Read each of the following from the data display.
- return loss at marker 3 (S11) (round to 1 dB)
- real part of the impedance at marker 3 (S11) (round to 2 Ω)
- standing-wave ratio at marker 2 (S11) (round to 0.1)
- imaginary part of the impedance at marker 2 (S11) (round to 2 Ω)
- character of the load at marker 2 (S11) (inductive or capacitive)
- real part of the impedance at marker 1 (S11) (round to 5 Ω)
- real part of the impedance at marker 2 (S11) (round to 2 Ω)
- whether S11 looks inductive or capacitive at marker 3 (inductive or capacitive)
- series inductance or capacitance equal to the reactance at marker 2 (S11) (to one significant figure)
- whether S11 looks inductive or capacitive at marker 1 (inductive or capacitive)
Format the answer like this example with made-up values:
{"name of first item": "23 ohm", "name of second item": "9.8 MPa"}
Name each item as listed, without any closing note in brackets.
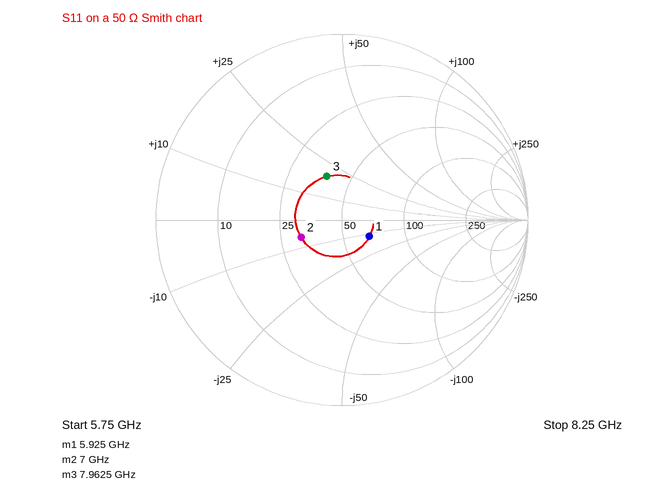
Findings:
{"return loss at marker 3 (S11)": "12 dB", "real part of the impedance at marker 3 (S11)": "38 Ω", "standing-wave ratio at marker 2 (S11)": "1.6", "imaginary part of the impedance at marker 2 (S11)": "-6 Ω", "character of the load at marker 2 (S11)": "capacitive", "real part of the impedance at marker 1 (S11)": "65 Ω", "real part of the impedance at marker 2 (S11)": "32 Ω", "whether S11 looks inductive or capacitive at marker 3": "inductive", "series inductance or capacitance equal to the reactance at marker 2 (S11)": "4 pF", "whether S11 looks inductive or capacitive at marker 1": "capacitive"}
